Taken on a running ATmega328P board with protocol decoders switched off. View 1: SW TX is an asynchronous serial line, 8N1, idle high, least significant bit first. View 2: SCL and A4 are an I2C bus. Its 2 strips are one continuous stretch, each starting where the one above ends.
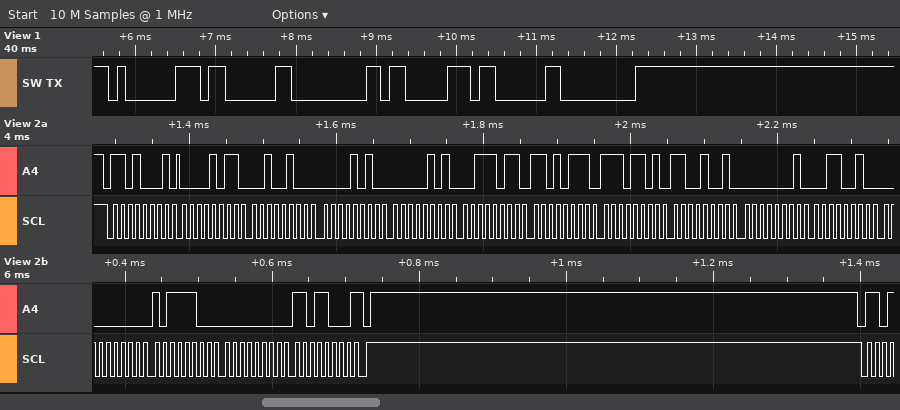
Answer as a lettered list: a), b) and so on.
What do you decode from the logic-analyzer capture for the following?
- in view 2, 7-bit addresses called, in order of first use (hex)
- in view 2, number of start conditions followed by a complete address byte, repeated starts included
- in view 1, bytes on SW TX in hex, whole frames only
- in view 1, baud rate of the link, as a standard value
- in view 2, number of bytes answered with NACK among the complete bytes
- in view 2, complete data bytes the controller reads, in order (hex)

a) 0x68
b) 1
c) 81 03 00 83 03 00
d) 9600 baud
e) 1
f) 0B 24 0A 05 3B D7 ED C9 01 32 00 BC 00 D8
